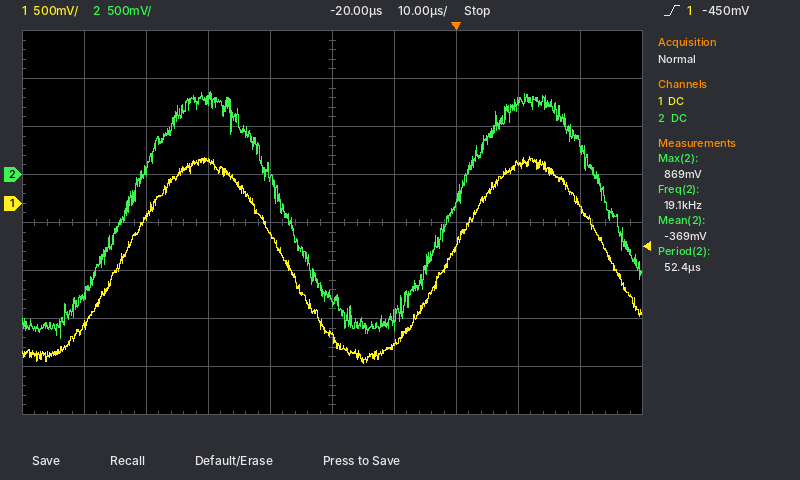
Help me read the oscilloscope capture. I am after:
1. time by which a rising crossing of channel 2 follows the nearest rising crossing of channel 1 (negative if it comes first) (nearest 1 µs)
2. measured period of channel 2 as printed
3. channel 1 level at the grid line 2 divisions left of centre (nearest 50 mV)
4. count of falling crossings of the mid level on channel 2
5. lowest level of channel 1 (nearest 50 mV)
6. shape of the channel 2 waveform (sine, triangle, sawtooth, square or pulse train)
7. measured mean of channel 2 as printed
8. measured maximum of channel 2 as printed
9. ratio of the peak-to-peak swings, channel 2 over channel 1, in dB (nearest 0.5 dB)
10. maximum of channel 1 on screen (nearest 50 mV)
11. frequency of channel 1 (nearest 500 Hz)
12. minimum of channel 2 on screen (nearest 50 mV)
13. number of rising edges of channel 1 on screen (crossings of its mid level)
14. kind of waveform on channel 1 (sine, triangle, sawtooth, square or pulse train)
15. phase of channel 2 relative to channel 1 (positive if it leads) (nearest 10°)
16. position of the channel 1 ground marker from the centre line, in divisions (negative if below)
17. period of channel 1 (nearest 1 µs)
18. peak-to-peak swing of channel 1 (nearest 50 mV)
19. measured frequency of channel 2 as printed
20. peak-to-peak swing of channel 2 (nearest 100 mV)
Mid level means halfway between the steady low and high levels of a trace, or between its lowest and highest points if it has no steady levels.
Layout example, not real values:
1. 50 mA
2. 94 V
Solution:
1. 0 µs
2. 52.4 µs
3. 450 mV
4. 2
5. -1.65 V
6. sine
7. -369 mV
8. 869 mV
9. 1.5 dB
10. 500 mV
11. 19.0 kHz
12. -1.70 V
13. 2
14. sine
15. 0°
16. +0.4 div
17. 53 µs
18. 2.15 V
19. 19.1 kHz
20. 2.60 V
